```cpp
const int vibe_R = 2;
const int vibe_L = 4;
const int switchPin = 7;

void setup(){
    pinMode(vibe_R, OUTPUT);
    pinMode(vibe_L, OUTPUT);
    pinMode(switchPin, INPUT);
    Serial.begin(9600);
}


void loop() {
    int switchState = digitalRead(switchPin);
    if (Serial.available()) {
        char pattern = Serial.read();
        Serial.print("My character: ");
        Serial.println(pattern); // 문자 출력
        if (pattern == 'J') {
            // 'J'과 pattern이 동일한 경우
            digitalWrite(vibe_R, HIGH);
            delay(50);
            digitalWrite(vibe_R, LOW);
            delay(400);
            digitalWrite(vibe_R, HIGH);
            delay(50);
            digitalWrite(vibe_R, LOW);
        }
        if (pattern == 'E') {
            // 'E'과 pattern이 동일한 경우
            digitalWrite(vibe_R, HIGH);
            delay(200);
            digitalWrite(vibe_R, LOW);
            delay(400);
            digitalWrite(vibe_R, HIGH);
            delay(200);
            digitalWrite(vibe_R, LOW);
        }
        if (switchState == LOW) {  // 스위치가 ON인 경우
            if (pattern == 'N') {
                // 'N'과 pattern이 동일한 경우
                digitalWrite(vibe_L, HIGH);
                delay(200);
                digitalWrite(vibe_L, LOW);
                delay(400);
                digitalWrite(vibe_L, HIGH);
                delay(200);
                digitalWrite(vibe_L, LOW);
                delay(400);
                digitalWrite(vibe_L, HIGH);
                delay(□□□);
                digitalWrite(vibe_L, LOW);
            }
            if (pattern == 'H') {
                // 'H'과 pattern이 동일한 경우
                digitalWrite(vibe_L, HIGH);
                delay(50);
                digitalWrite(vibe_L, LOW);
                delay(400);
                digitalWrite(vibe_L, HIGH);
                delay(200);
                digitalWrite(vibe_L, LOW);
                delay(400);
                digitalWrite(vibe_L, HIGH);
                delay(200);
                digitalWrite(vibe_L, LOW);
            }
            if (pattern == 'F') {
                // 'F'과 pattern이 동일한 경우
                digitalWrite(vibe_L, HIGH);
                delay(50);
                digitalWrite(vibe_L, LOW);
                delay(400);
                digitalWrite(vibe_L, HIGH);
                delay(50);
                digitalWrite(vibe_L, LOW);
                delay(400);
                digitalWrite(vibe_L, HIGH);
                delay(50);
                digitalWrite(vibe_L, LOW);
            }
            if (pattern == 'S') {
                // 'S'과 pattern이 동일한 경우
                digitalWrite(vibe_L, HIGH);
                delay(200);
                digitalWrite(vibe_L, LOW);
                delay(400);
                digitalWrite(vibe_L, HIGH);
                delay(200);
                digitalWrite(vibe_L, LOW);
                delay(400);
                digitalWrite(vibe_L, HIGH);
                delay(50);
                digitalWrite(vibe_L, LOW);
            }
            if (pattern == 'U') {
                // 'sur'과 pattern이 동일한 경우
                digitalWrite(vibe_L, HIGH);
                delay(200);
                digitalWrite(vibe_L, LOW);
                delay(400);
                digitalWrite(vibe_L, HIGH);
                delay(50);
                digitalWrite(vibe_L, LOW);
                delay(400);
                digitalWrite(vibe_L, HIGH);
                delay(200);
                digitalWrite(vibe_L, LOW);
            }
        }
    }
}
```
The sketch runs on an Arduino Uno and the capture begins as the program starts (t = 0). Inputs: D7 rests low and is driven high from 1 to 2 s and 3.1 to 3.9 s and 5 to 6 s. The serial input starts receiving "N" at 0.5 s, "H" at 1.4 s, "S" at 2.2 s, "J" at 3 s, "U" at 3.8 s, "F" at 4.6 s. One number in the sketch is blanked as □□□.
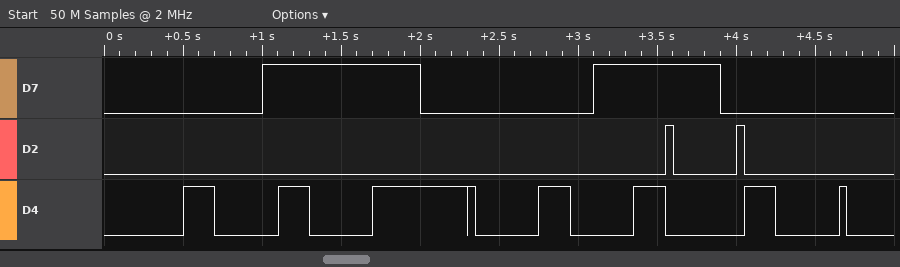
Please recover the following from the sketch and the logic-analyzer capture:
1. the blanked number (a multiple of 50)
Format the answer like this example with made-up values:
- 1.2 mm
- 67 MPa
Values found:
- 600
